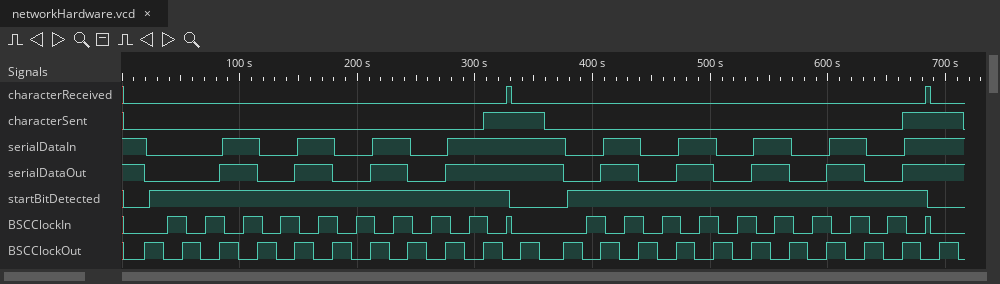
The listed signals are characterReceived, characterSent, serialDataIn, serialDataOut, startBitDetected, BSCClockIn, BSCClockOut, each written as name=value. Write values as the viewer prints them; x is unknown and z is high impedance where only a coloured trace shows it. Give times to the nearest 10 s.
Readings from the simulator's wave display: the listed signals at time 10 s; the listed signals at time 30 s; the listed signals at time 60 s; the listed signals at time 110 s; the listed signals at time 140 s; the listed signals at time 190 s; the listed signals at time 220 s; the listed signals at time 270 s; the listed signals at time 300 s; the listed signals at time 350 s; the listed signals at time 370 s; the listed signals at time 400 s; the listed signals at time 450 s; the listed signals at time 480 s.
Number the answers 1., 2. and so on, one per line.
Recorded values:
1. characterReceived=0, characterSent=0, serialDataIn=1, serialDataOut=1, startBitDetected=0, BSCClockIn=0, BSCClockOut=0
2. characterReceived=0, characterSent=0, serialDataIn=0, serialDataOut=0, startBitDetected=1, BSCClockIn=0, BSCClockOut=1
3. characterReceived=0, characterSent=0, serialDataIn=0, serialDataOut=0, startBitDetected=1, BSCClockIn=0, BSCClockOut=1
4. characterReceived=0, characterSent=0, serialDataIn=1, serialDataOut=1, startBitDetected=1, BSCClockIn=1, BSCClockOut=0
5. characterReceived=0, characterSent=0, serialDataIn=0, serialDataOut=0, startBitDetected=1, BSCClockIn=1, BSCClockOut=0
6. characterReceived=0, characterSent=0, serialDataIn=0, serialDataOut=0, startBitDetected=1, BSCClockIn=0, BSCClockOut=1
7. characterReceived=0, characterSent=0, serialDataIn=1, serialDataOut=1, startBitDetected=1, BSCClockIn=0, BSCClockOut=1
8. characterReceived=0, characterSent=0, serialDataIn=0, serialDataOut=0, startBitDetected=1, BSCClockIn=1, BSCClockOut=0
9. characterReceived=0, characterSent=0, serialDataIn=1, serialDataOut=1, startBitDetected=1, BSCClockIn=1, BSCClockOut=0
10. characterReceived=0, characterSent=1, serialDataIn=1, serialDataOut=1, startBitDetected=0, BSCClockIn=0, BSCClockOut=1
11. characterReceived=0, characterSent=0, serialDataIn=1, serialDataOut=1, startBitDetected=0, BSCClockIn=0, BSCClockOut=0
12. characterReceived=0, characterSent=0, serialDataIn=0, serialDataOut=0, startBitDetected=1, BSCClockIn=1, BSCClockOut=0
13. characterReceived=0, characterSent=0, serialDataIn=0, serialDataOut=0, startBitDetected=1, BSCClockIn=0, BSCClockOut=1
14. characterReceived=0, characterSent=0, serialDataIn=1, serialDataOut=1, startBitDetected=1, BSCClockIn=0, BSCClockOut=1
